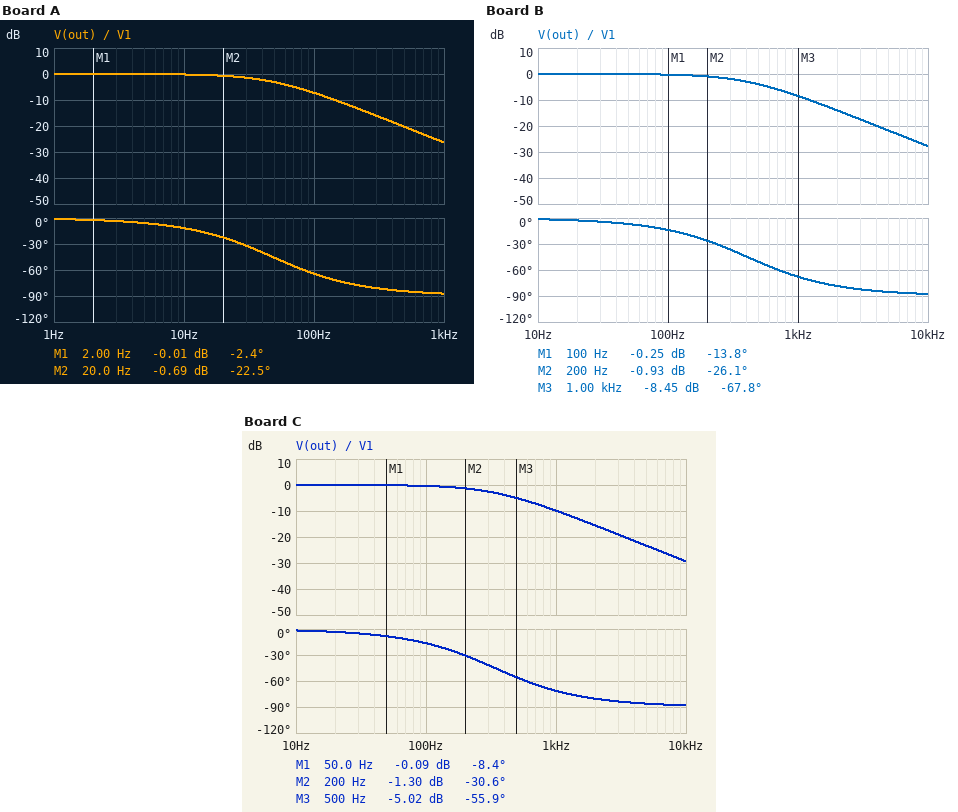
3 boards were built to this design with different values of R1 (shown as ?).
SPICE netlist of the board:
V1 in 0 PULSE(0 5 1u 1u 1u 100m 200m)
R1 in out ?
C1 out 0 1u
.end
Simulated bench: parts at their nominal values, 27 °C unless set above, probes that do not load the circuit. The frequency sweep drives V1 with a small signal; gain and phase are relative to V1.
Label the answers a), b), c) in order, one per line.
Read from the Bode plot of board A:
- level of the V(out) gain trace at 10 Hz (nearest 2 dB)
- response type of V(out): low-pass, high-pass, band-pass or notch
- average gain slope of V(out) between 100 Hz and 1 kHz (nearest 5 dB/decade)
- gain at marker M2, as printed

a) 0 dB
b) low-pass
c) -20 dB/decade
d) -0.69 dB
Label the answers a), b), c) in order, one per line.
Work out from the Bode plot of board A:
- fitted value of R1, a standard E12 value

a) 3.3 kΩ
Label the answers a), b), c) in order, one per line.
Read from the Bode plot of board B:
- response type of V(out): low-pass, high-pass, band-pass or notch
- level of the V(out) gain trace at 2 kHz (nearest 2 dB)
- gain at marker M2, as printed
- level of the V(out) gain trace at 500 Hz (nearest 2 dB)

a) low-pass
b) -14 dB
c) -0.93 dB
d) -4 dB
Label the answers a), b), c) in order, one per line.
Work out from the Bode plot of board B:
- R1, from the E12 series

a) 390 Ω
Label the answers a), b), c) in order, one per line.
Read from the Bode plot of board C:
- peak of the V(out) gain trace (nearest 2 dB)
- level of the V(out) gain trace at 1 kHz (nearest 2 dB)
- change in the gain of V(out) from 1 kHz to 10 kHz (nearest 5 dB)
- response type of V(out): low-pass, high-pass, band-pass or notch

a) 0 dB
b) -10 dB
c) -20 dB
d) low-pass
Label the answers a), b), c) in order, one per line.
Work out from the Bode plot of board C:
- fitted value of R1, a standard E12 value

a) 470 Ω
